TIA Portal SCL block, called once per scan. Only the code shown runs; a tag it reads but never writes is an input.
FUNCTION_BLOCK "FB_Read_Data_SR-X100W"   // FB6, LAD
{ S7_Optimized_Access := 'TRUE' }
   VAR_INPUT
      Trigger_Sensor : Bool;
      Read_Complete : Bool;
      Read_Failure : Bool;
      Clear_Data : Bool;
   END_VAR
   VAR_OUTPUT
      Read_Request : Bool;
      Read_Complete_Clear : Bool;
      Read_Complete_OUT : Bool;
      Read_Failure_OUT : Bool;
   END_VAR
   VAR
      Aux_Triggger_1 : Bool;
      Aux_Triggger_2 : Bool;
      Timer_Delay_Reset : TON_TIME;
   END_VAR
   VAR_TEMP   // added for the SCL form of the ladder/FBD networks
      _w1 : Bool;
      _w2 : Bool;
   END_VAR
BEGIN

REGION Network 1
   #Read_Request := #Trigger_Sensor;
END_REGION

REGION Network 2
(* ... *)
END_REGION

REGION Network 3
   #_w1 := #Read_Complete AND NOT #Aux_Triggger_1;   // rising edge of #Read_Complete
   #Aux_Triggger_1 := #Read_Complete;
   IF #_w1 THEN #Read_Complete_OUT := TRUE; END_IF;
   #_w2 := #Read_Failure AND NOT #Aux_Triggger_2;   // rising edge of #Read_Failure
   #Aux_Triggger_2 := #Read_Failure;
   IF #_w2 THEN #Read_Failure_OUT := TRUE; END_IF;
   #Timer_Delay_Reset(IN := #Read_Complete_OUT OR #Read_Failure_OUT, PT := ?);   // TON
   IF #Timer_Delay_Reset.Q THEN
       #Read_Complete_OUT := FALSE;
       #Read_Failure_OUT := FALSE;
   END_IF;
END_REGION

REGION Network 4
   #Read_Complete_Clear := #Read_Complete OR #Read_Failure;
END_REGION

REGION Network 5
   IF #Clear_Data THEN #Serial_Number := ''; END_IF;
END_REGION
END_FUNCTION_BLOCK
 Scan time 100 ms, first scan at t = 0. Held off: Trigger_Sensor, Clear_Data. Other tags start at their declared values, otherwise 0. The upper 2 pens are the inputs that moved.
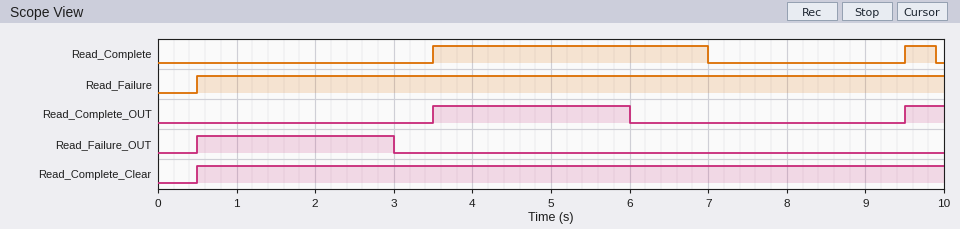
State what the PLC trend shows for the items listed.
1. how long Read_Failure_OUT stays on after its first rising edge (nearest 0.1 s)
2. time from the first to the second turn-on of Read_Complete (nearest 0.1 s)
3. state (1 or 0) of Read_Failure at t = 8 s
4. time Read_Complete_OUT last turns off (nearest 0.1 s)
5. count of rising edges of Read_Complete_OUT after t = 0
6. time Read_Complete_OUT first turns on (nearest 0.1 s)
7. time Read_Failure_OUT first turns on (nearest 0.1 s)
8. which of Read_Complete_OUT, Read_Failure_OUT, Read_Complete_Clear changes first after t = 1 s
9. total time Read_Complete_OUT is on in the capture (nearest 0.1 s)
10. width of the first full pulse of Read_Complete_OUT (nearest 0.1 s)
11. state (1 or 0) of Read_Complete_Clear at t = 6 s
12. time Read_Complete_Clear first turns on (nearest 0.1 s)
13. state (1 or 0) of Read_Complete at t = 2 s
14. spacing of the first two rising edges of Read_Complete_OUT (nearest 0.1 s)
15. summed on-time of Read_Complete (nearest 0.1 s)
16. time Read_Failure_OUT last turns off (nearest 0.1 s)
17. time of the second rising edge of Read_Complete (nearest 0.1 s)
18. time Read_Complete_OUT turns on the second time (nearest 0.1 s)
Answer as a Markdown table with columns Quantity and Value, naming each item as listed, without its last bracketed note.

| Quantity | Value |
|---|---|
| how long Read_Failure_OUT stays on after its first rising edge | 2.5 s |
| time from the first to the second turn-on of Read_Complete | 6.0 s |
| state (1 or 0) of Read_Failure at t = 8 s | 1 |
| time Read_Complete_OUT last turns off | 6.0 s |
| count of rising edges of Read_Complete_OUT after t = 0 | 2 |
| time Read_Complete_OUT first turns on | 3.5 s |
| time Read_Failure_OUT first turns on | 0.5 s |
| which of Read_Complete_OUT, Read_Failure_OUT, Read_Complete_Clear changes first after t = 1 s | Read_Failure_OUT |
| total time Read_Complete_OUT is on in the capture | 3.0 s |
| width of the first full pulse of Read_Complete_OUT | 2.5 s |
| state (1 or 0) of Read_Complete_Clear at t = 6 s | 1 |
| time Read_Complete_Clear first turns on | 0.5 s |
| state (1 or 0) of Read_Complete at t = 2 s | 0 |
| spacing of the first two rising edges of Read_Complete_OUT | 6.0 s |
| summed on-time of Read_Complete | 3.9 s |
| time Read_Failure_OUT last turns off | 3.0 s |
| time of the second rising edge of Read_Complete | 9.5 s |
| time Read_Complete_OUT turns on the second time | 9.5 s |
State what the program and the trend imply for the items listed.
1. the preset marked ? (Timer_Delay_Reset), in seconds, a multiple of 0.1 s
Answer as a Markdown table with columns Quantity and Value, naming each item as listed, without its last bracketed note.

| Quantity | Value |
|---|---|
| the preset marked ? (Timer_Delay_Reset), in seconds, a multiple of 0.1 s | 2.5 s |
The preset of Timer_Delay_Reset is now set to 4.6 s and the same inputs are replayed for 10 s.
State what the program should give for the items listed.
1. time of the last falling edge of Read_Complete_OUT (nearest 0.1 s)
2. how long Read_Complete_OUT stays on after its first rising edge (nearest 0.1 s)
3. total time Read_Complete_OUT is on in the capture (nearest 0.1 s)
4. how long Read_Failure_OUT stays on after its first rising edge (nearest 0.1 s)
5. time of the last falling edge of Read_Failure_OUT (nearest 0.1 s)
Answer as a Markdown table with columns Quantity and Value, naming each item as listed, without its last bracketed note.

| Quantity | Value |
|---|---|
| time of the last falling edge of Read_Complete_OUT | 5.1 s |
| how long Read_Complete_OUT stays on after its first rising edge | 1.6 s |
| total time Read_Complete_OUT is on in the capture | 2.1 s |
| how long Read_Failure_OUT stays on after its first rising edge | 4.6 s |
| time of the last falling edge of Read_Failure_OUT | 5.1 s |
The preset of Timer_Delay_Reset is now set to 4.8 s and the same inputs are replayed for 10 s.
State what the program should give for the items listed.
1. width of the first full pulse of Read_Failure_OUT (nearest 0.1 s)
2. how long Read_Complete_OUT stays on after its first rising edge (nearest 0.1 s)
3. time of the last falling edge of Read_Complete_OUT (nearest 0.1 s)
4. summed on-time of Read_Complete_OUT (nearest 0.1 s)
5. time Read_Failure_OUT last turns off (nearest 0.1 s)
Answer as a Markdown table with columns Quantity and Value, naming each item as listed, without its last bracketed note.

| Quantity | Value |
|---|---|
| width of the first full pulse of Read_Failure_OUT | 4.8 s |
| how long Read_Complete_OUT stays on after its first rising edge | 1.8 s |
| time of the last falling edge of Read_Complete_OUT | 5.3 s |
| summed on-time of Read_Complete_OUT | 2.3 s |
| time Read_Failure_OUT last turns off | 5.3 s |
